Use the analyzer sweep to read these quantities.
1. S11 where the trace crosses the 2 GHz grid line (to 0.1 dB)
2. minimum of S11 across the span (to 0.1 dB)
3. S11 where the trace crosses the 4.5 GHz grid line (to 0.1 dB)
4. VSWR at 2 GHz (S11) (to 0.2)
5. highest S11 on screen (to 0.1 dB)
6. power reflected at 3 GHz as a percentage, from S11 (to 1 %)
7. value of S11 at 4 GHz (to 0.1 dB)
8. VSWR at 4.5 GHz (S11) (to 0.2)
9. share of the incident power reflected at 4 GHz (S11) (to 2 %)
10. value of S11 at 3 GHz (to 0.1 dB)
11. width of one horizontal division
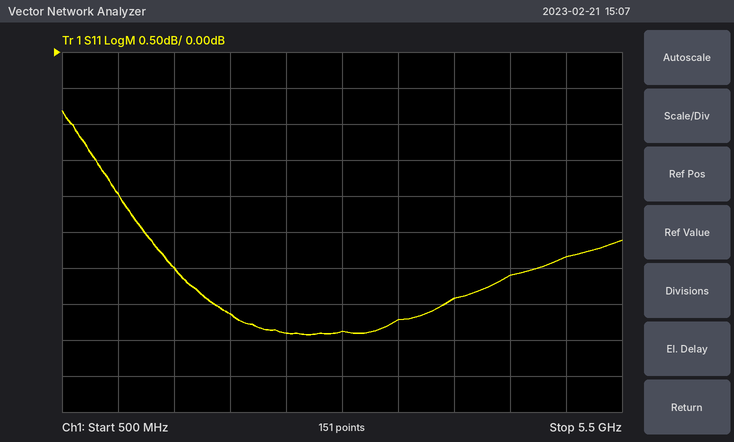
-3.6 dB
-3.9 dB
-3.1 dB
4.8
-0.8 dB
41 %
-3.4 dB
5.6
46 %
-3.9 dB
500 MHz
